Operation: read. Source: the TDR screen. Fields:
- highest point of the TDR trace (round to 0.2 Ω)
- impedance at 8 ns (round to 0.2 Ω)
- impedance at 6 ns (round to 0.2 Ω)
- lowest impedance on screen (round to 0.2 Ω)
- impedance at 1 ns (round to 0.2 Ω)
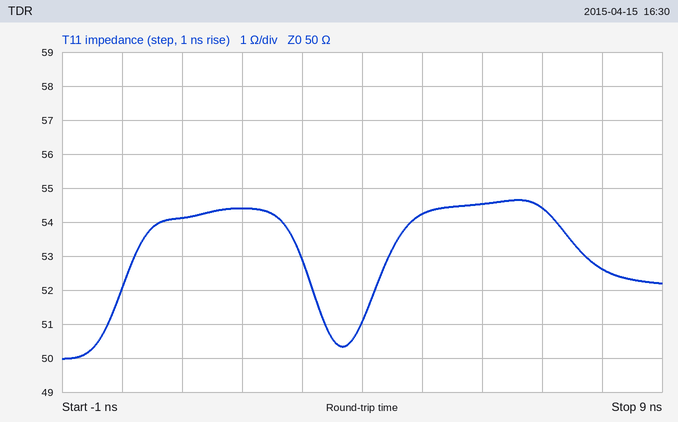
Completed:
54.6 Ω
52.6 Ω
54.6 Ω
50.0 Ω
54.2 Ω
